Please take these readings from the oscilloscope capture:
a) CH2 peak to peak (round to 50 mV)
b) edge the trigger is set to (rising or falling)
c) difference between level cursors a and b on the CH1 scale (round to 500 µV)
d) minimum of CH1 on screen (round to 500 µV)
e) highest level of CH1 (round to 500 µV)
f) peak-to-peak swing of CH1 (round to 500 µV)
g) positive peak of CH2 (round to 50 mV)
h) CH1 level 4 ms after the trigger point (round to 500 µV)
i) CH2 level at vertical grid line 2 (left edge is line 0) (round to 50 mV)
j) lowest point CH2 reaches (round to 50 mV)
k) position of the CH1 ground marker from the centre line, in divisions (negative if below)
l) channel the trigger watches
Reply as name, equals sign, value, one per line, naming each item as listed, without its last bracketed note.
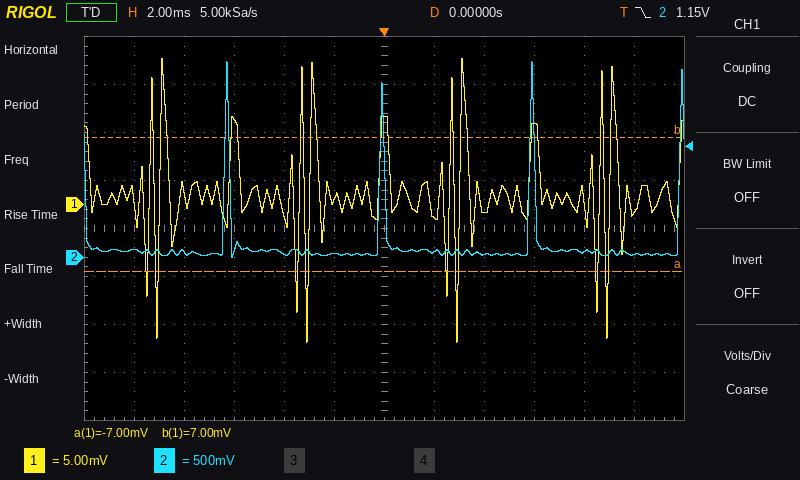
CH2 peak to peak = 2.05 V
edge the trigger is set to = falling
difference between level cursors a and b on the CH1 scale = 14.0 mV
minimum of CH1 on screen = -14.5 mV
highest level of CH1 = 15.0 mV
peak-to-peak swing of CH1 = 29.5 mV
positive peak of CH2 = 2.05 V
CH1 level 4 ms after the trigger point = -500 µV
CH2 level at vertical grid line 2 (left edge is line 0) = 50 mV
lowest point CH2 reaches = 0 mV
position of the CH1 ground marker from the centre line, in divisions = +0.5 div
channel the trigger watches = CH2
